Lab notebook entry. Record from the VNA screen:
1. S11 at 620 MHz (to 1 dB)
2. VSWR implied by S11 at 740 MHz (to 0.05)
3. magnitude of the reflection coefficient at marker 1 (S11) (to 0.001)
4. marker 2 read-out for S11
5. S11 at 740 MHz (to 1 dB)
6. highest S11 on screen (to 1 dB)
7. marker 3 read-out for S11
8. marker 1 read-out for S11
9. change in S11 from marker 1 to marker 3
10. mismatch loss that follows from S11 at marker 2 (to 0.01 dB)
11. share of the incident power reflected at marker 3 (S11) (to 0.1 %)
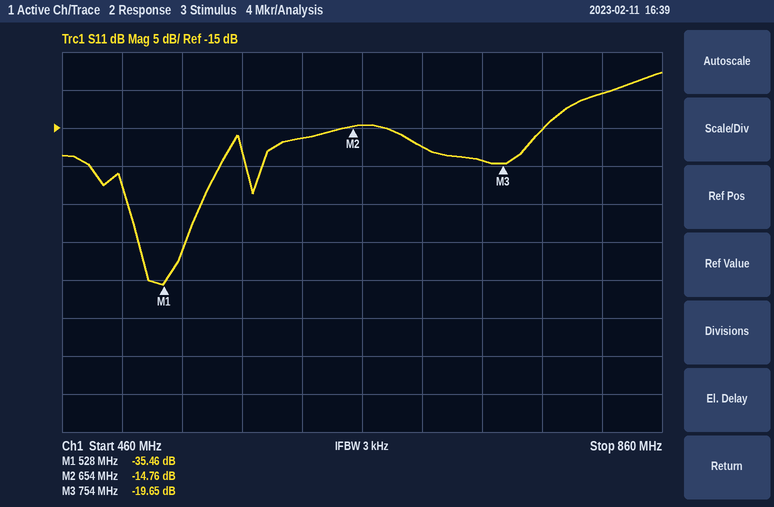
-16 dB
1.25
0.017
-14.76 dB
-19 dB
-8 dB
-19.65 dB
-35.46 dB
15.81 dB
0.15 dB
1.1 %
